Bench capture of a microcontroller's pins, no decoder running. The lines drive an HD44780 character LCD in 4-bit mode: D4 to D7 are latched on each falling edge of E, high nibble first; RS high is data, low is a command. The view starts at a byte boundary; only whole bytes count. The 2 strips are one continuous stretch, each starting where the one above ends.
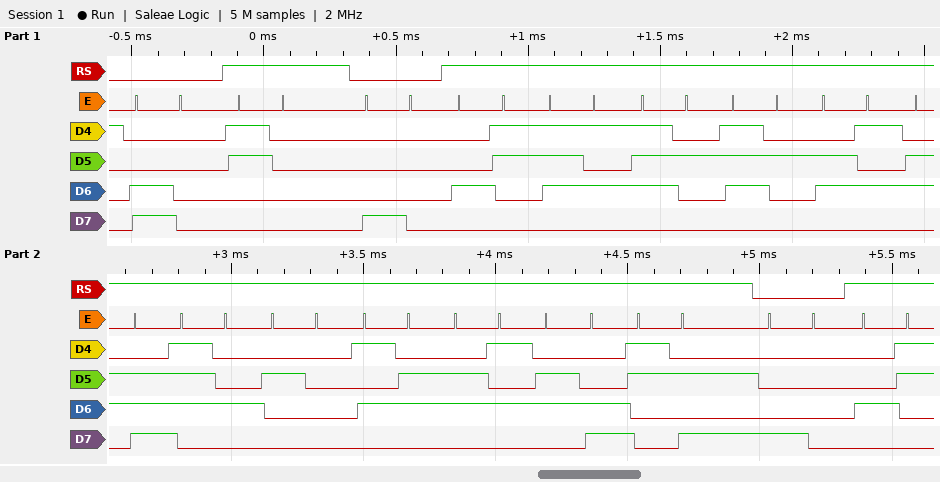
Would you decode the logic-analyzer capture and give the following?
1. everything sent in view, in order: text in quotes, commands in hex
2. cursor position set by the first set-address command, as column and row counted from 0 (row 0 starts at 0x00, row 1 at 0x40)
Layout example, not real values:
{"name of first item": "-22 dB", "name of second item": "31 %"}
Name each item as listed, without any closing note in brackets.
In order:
{"everything sent in view, in order: text in quotes, commands in hex": "0xC0 \"0\" 0x80 \"Current Vel:\" 0x80 \"C\"", "cursor position set by the first set-address command, as column and row counted from 0": "column 0, row 1"}
